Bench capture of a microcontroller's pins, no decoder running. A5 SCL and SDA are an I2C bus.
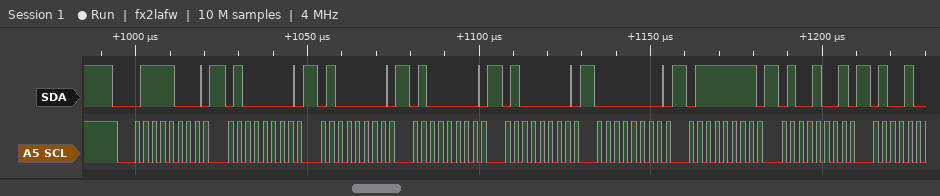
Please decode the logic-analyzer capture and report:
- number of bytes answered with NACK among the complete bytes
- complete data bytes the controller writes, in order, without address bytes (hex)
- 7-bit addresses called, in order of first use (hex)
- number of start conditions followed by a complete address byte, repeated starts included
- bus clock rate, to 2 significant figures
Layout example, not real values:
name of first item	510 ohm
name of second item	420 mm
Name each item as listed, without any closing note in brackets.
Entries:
number of bytes answered with NACK among the complete bytes	0
complete data bytes the controller writes, in order, without address bytes	40 40 40 40 00 7F 49
7-bit addresses called, in order of first use	0x3C
number of start conditions followed by a complete address byte, repeated starts included	1
bus clock rate, to 2 significant figures	400 kHz
